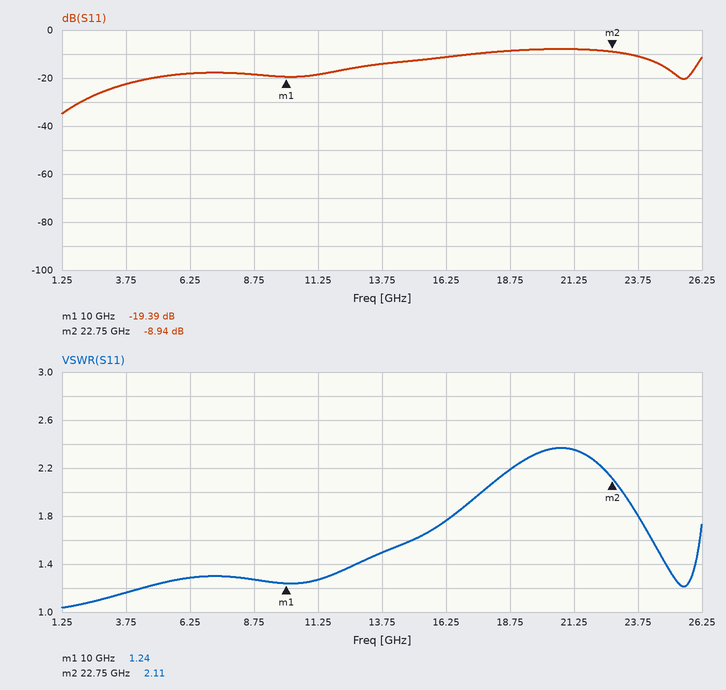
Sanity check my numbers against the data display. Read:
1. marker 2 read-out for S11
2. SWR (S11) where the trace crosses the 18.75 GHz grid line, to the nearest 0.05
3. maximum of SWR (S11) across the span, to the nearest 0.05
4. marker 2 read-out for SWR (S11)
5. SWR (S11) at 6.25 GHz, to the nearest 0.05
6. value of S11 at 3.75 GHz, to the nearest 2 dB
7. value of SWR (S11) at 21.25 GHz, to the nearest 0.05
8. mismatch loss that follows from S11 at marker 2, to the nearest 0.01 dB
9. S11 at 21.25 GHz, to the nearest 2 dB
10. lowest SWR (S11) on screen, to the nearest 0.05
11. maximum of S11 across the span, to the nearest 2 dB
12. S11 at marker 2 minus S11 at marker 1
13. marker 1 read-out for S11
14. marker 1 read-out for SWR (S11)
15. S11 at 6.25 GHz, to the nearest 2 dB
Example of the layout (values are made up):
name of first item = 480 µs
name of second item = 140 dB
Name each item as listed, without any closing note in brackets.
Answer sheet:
marker 2 read-out for S11 = -8.94 dB
SWR (S11) where the trace crosses the 18.75 GHz grid line, to the nearest 0.05 = 2.20
maximum of SWR (S11) across the span, to the nearest 0.05 = 2.35
marker 2 read-out for SWR = 2.11
SWR (S11) at 6.25 GHz, to the nearest 0.05 = 1.30
value of S11 at 3.75 GHz, to the nearest 2 dB = -22 dB
value of SWR (S11) at 21.25 GHz, to the nearest 0.05 = 2.35
mismatch loss that follows from S11 at marker 2, to the nearest 0.01 dB = 0.59 dB
S11 at 21.25 GHz, to the nearest 2 dB = -8 dB
lowest SWR (S11) on screen, to the nearest 0.05 = 1.05
maximum of S11 across the span, to the nearest 2 dB = -8 dB
S11 at marker 2 minus S11 at marker 1 = 10.45 dB
marker 1 read-out for S11 = -19.39 dB
marker 1 read-out for SWR = 1.24
S11 at 6.25 GHz, to the nearest 2 dB = -18 dB
